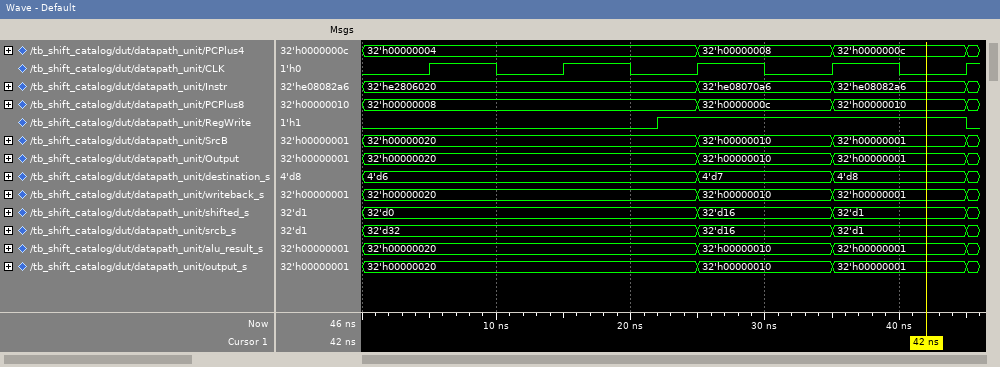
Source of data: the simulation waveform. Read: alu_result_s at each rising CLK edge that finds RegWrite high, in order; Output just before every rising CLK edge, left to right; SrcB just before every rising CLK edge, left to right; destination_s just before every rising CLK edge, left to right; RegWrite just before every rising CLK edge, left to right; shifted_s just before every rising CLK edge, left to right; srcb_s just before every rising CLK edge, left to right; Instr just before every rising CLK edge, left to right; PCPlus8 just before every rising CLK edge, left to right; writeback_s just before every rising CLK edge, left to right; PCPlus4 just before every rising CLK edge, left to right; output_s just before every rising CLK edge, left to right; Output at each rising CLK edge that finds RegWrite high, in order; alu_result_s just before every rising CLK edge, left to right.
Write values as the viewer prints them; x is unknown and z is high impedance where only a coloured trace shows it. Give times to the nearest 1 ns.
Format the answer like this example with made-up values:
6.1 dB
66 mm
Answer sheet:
32'h00000020, 32'h00000010, 32'h00000001
32'h00000020, 32'h00000020, 32'h00000020, 32'h00000010, 32'h00000001
32'h00000020, 32'h00000020, 32'h00000020, 32'h00000010, 32'h00000001
4'd6, 4'd6, 4'd6, 4'd7, 4'd8
0 0 1 1 1
32'd0, 32'd0, 32'd0, 32'd16, 32'd1
32'd32, 32'd32, 32'd32, 32'd16, 32'd1
32'he2806020, 32'he2806020, 32'he2806020, 32'he08070a6, 32'he08082a6
32'h00000008, 32'h00000008, 32'h00000008, 32'h0000000c, 32'h00000010
32'h00000020, 32'h00000020, 32'h00000020, 32'h00000010, 32'h00000001
32'h00000004, 32'h00000004, 32'h00000004, 32'h00000008, 32'h0000000c
32'h00000020, 32'h00000020, 32'h00000020, 32'h00000010, 32'h00000001
32'h00000020, 32'h00000010, 32'h00000001
32'h00000020, 32'h00000020, 32'h00000020, 32'h00000010, 32'h00000001
